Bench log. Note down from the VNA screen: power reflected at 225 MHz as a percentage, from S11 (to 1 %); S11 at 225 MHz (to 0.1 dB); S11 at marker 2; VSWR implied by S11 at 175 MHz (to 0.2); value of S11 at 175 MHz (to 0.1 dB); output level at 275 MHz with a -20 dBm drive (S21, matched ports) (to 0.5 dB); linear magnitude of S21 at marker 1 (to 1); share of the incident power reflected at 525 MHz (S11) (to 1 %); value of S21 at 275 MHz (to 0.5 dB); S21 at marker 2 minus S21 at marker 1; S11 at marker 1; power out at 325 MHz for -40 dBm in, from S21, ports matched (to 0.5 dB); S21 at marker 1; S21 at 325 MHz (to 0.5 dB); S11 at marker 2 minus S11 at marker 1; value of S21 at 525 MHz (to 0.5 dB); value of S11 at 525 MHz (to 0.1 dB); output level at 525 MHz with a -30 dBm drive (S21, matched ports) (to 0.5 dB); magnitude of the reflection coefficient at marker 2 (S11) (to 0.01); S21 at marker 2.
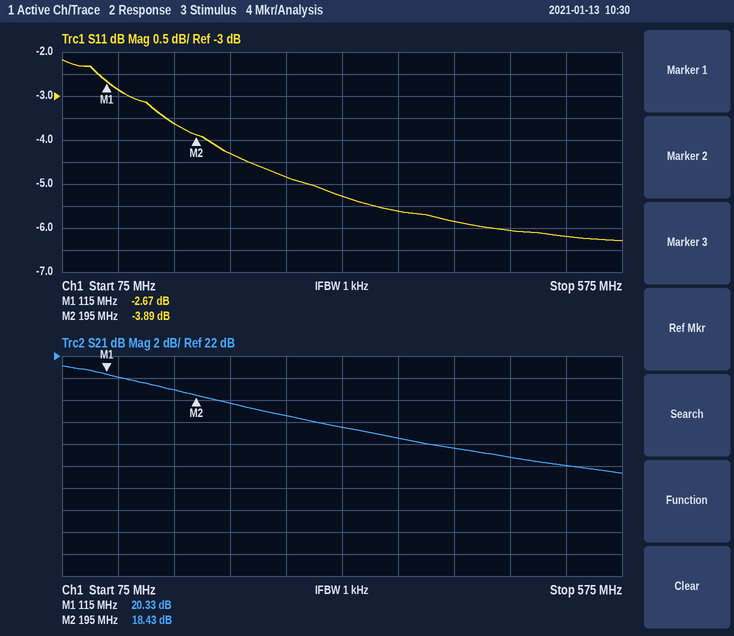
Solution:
37 %
-4.3 dB
-3.89 dB
4.8
-3.6 dB
-3.5 dBm
10
24 %
16.5 dB
-1.90 dB
-2.67 dB
-24.5 dBm
20.33 dB
15.5 dB
-1.22 dB
12.0 dB
-6.2 dB
-18.0 dBm
0.64
18.43 dB
